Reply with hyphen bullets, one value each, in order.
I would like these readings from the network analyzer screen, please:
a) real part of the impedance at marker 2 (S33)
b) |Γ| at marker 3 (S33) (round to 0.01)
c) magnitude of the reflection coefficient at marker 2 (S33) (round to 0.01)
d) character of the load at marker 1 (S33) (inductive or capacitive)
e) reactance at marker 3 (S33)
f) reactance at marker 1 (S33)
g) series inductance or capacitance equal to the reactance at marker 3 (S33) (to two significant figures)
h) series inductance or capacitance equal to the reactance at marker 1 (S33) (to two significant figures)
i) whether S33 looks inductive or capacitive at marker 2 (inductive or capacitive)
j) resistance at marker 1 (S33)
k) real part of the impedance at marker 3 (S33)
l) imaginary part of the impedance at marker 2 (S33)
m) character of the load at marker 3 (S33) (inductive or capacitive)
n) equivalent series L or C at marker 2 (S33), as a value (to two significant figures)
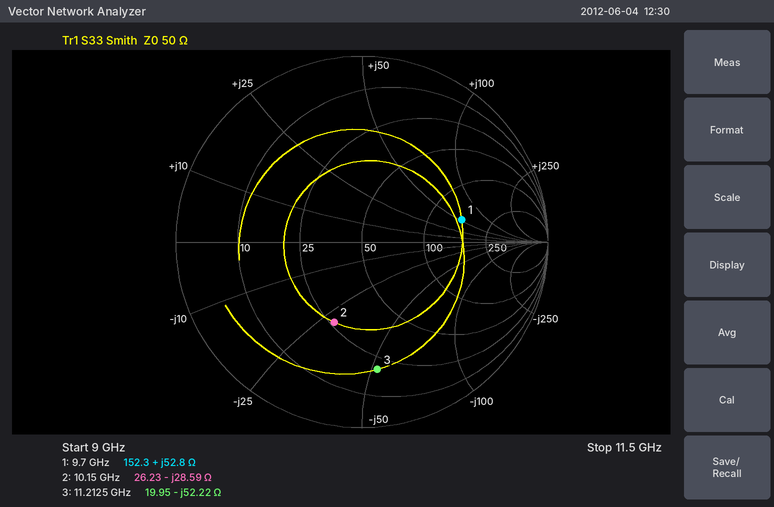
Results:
- 26.23 Ω
- 0.69
- 0.46
- inductive
- -52.22 Ω
- +52.8 Ω
- 270 fF
- 870 pH
- capacitive
- 152.3 Ω
- 19.95 Ω
- -28.59 Ω
- capacitive
- 550 fF
